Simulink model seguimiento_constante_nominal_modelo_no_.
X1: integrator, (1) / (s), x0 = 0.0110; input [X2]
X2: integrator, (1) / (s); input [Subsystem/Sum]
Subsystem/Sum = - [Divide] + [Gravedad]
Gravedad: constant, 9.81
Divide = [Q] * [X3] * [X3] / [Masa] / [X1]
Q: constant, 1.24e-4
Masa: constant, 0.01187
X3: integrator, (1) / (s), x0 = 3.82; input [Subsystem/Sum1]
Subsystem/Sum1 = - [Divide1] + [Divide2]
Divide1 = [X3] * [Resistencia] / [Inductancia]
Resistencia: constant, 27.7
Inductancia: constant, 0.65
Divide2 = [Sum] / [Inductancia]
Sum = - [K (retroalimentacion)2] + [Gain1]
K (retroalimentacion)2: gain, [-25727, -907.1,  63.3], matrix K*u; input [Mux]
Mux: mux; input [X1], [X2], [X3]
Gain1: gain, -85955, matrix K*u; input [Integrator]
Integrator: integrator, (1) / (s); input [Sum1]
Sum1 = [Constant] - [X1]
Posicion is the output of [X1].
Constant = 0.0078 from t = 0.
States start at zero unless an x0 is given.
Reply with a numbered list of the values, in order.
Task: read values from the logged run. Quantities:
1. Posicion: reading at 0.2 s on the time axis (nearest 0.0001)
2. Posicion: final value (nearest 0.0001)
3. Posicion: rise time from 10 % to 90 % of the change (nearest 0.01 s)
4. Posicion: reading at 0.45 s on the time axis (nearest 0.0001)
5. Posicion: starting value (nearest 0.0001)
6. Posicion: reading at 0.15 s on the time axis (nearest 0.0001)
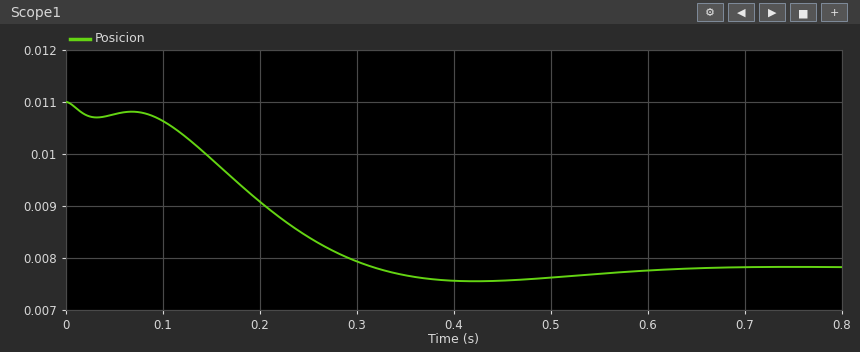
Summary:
1. 0.0091
2. 0.0078
3. 0.18 s
4. 0.0076
5. 0.0110
6. 0.0099
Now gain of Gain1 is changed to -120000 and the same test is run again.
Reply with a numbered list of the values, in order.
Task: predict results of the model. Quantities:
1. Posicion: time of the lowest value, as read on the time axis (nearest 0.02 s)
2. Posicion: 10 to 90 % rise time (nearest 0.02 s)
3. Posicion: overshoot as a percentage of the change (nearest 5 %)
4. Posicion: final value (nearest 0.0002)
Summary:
1. 0.32 s
2. 0.14 s
3. 15 %
4. 0.0078
